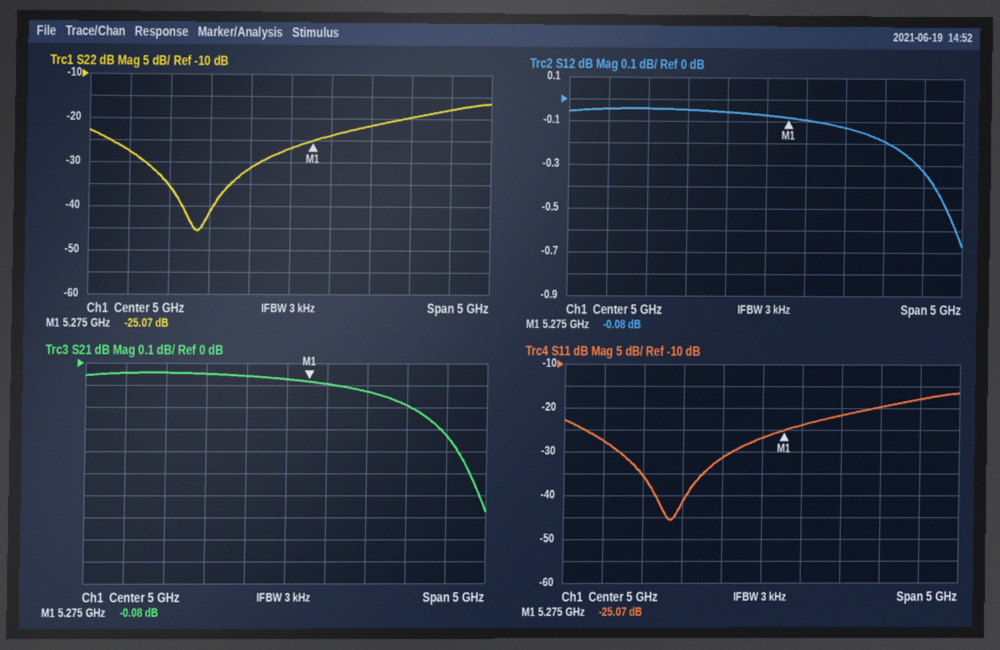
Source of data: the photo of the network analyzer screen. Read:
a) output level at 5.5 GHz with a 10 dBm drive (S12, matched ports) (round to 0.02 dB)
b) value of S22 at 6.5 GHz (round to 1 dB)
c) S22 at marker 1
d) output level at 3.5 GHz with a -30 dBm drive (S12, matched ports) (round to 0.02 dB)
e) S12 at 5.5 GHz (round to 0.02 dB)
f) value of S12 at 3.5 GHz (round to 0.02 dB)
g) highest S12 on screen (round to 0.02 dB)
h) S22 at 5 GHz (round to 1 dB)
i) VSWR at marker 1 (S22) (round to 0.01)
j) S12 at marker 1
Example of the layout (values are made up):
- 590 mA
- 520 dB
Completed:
- 9.90 dBm
- -20 dB
- -25.07 dB
- -30.04 dBm
- -0.10 dB
- -0.04 dB
- -0.04 dB
- -27 dB
- 1.12
- -0.08 dB
